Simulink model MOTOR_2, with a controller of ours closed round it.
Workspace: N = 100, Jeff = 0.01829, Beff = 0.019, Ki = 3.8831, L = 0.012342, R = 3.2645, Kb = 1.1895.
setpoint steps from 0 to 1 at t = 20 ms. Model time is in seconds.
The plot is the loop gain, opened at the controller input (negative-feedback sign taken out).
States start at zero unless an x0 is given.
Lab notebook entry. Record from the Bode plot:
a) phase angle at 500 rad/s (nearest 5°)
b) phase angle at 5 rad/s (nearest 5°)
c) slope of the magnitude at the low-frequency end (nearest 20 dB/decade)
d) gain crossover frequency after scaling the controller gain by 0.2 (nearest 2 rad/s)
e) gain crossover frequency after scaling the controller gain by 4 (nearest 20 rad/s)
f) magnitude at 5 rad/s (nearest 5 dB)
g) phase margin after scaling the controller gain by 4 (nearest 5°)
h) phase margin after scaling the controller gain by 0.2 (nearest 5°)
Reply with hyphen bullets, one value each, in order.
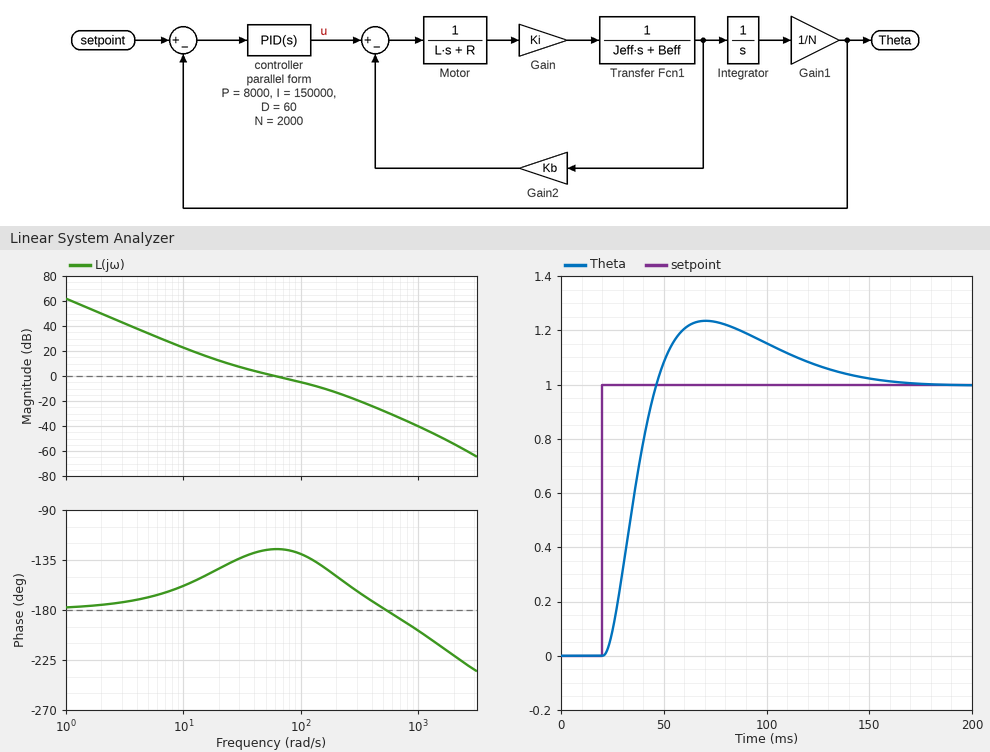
- -180°
- -170°
- -40 dB/decade
- 18 rad/s
- 180 rad/s
- 35 dB
- 35°
- 35°
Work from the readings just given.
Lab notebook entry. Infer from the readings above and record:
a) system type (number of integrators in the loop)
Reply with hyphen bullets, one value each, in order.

- 2
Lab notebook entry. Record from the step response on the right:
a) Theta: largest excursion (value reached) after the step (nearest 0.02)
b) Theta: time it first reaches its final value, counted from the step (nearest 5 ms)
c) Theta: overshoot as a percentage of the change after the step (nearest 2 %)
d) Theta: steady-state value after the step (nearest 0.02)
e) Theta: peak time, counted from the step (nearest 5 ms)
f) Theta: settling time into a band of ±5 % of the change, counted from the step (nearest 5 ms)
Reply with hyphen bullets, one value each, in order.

- 1.24
- 25 ms
- 24 %
- 1.00
- 50 ms
- 115 ms
